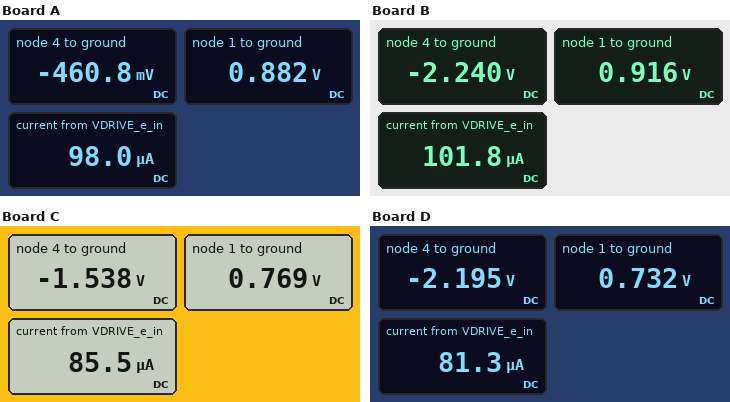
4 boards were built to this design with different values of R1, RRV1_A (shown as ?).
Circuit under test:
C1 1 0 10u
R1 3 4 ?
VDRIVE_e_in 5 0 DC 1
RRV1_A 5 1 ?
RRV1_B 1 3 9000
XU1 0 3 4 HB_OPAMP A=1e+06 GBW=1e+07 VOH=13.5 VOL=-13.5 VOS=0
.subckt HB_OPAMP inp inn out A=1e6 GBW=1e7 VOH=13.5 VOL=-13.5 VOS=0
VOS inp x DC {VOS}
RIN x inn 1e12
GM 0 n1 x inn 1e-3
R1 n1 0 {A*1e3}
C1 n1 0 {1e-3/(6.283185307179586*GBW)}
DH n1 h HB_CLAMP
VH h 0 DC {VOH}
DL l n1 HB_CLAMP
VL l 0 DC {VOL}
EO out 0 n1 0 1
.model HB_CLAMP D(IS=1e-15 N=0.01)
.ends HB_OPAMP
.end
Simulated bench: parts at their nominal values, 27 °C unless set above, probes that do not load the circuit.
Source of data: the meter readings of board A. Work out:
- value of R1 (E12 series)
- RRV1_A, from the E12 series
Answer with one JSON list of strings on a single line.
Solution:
["4.7 kΩ", "1.2 kΩ"]
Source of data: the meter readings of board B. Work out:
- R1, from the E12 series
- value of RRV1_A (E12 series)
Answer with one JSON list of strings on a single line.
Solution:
["22 kΩ", "820 Ω"]
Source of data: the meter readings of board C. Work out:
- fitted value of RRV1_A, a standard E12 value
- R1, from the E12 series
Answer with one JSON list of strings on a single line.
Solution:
["2.7 kΩ", "18 kΩ"]
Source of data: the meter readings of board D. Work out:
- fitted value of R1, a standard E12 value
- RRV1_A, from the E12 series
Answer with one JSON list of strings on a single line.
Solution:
["27 kΩ", "3.3 kΩ"]
